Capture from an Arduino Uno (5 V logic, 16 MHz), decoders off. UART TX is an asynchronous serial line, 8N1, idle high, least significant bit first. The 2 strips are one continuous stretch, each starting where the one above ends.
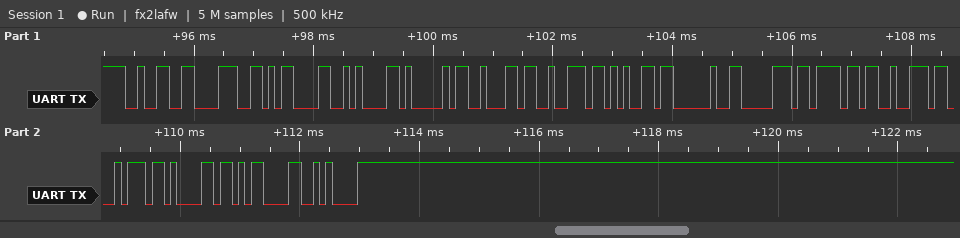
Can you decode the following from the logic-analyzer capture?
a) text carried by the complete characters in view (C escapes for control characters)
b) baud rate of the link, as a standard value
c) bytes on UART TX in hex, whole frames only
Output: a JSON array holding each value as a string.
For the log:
["\"28\\r\\nAbre porta\\r\\n\"", "9600 baud", "32 38 0D 0A 41 62 72 65 20 70 6F 72 74 61 0D 0A"]
